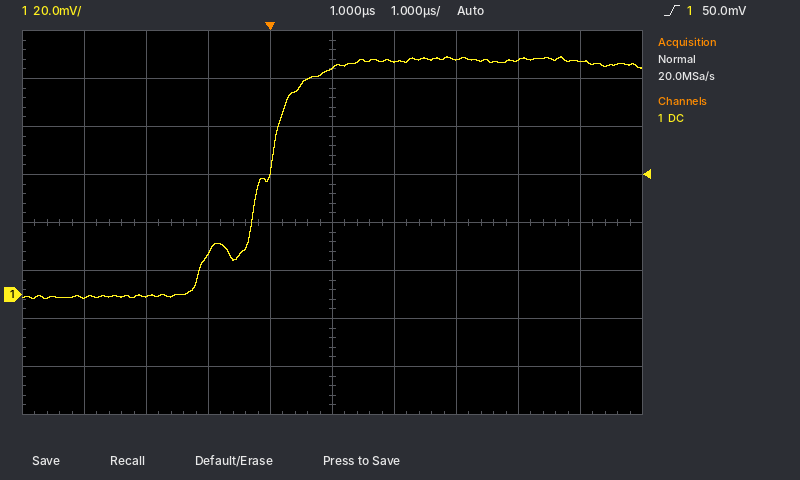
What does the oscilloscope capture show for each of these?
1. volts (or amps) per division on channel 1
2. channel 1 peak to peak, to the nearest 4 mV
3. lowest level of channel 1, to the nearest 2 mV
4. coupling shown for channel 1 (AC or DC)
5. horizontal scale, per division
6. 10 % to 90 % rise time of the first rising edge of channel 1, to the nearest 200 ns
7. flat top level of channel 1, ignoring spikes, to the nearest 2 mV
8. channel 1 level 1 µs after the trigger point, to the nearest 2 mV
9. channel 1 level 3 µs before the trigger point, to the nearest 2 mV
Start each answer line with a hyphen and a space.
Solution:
- 20 mV
- 100 mV
- -2 mV
- DC
- 1 µs
- 1.6 µs
- 98 mV
- 94 mV
- -2 mV
